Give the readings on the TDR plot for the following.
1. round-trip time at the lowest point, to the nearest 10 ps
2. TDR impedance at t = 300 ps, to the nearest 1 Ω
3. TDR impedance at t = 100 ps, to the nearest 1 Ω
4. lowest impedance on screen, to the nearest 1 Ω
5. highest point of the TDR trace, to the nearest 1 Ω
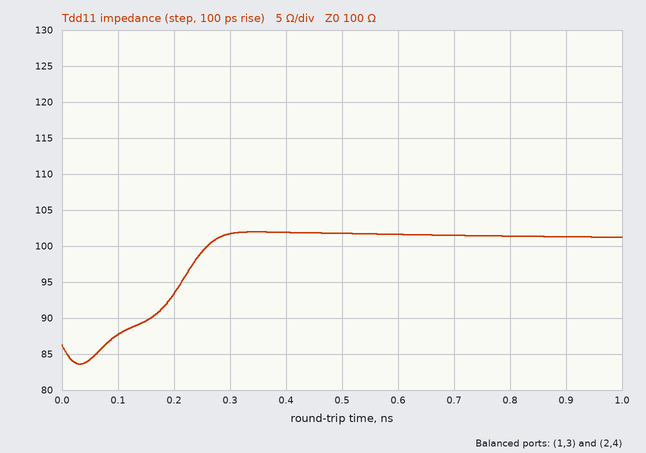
30 ps
102 Ω
88 Ω
84 Ω
102 Ω
